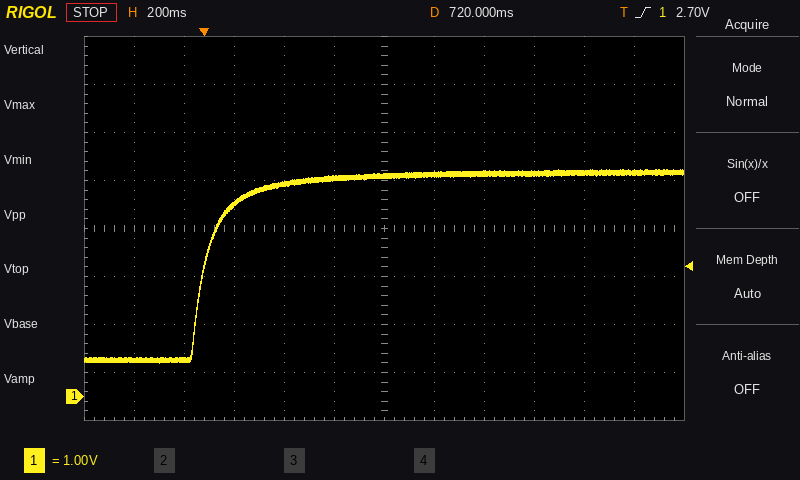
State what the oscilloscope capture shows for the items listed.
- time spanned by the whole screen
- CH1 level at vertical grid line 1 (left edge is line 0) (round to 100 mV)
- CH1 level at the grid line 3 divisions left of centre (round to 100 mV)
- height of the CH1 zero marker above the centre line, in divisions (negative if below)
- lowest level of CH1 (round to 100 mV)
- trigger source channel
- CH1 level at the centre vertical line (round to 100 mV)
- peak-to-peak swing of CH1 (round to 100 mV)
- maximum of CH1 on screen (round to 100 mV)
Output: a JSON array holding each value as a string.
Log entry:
["2.4 s", "800 mV", "4.0 V", "-3.5 div", "700 mV", "CH1", "4.6 V", "4.0 V", "4.7 V"]
